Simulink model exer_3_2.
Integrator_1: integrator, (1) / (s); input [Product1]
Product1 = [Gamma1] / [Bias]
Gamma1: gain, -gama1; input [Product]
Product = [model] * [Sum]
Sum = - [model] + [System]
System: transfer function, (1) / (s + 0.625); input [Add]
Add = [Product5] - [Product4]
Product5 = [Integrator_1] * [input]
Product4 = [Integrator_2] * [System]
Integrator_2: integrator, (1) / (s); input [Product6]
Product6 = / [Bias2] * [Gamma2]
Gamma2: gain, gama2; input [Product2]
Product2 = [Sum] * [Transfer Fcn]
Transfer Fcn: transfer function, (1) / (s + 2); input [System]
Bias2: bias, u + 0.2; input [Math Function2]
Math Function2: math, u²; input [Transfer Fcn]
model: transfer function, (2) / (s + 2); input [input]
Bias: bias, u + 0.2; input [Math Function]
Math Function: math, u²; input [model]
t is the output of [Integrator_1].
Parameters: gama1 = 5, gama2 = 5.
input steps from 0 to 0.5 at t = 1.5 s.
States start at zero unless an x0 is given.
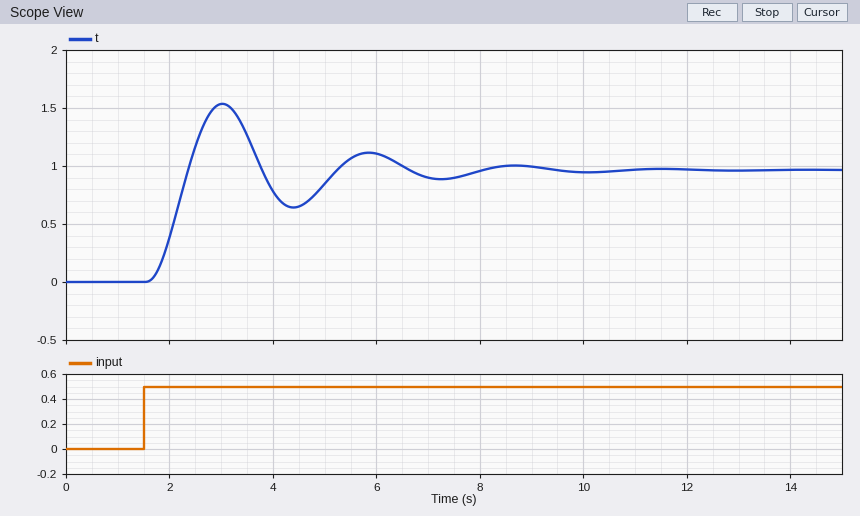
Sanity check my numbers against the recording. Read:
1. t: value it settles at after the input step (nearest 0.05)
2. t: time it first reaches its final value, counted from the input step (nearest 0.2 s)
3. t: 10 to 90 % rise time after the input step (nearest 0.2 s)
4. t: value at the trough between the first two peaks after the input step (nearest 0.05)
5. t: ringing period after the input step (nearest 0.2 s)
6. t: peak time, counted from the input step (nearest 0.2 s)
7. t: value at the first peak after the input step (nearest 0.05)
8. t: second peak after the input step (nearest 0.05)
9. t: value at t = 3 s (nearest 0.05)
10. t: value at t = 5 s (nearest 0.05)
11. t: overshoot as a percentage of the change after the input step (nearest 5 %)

0.95
0.8 s
0.6 s
0.65
2.8 s
1.6 s
1.55
1.10
1.55
0.85
60 %
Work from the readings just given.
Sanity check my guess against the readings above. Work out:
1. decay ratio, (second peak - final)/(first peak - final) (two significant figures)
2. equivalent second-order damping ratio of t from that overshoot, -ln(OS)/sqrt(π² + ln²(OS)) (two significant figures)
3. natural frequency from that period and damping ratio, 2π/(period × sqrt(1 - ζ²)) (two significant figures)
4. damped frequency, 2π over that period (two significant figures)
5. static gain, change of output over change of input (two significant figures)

0.25
0.16
2.3 rad/s
2.2 rad/s
1.9
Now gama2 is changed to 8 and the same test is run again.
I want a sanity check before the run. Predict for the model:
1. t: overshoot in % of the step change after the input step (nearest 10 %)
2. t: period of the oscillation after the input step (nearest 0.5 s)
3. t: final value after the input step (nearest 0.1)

50 %
2.5 s
1.0
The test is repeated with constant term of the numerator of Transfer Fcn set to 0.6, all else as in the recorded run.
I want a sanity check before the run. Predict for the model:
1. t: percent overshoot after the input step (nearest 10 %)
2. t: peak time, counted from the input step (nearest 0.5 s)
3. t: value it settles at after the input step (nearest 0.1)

70 %
1.5 s
0.9
